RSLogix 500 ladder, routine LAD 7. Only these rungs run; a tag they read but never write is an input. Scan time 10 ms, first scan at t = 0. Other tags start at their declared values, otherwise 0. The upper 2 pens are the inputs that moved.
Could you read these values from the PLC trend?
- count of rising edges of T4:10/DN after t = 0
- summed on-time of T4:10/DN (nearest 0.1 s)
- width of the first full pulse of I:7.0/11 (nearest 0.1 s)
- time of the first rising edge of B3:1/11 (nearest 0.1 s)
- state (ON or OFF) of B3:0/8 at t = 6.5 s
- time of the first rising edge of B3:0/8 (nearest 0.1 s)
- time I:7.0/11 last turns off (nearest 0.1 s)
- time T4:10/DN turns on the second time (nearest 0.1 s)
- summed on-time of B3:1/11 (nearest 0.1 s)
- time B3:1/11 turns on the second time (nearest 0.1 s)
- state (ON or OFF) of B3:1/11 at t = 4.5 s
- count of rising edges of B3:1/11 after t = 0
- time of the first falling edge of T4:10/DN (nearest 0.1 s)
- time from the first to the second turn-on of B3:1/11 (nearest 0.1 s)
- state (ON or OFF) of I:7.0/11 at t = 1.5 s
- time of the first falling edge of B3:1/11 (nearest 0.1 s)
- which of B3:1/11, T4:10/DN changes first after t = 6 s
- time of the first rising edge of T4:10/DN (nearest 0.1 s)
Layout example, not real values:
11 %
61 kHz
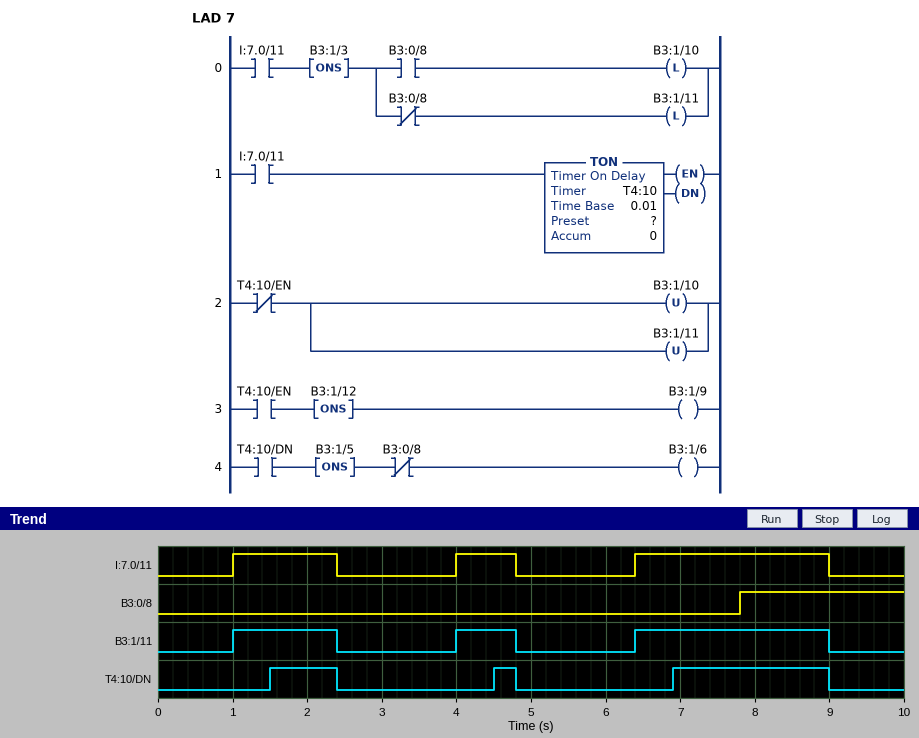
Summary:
3
3.3 s
1.4 s
1.0 s
OFF
7.8 s
9.0 s
4.5 s
4.8 s
4.0 s
ON
3
2.4 s
3.0 s
ON
2.4 s
B3:1/11
1.5 s
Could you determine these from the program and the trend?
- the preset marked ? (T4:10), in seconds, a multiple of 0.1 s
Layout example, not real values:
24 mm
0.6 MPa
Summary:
0.5 s
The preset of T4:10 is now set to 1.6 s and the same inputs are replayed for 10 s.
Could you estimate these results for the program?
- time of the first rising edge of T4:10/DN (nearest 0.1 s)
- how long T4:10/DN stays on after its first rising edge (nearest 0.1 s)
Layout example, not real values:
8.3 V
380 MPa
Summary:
8.0 s
1.0 s
